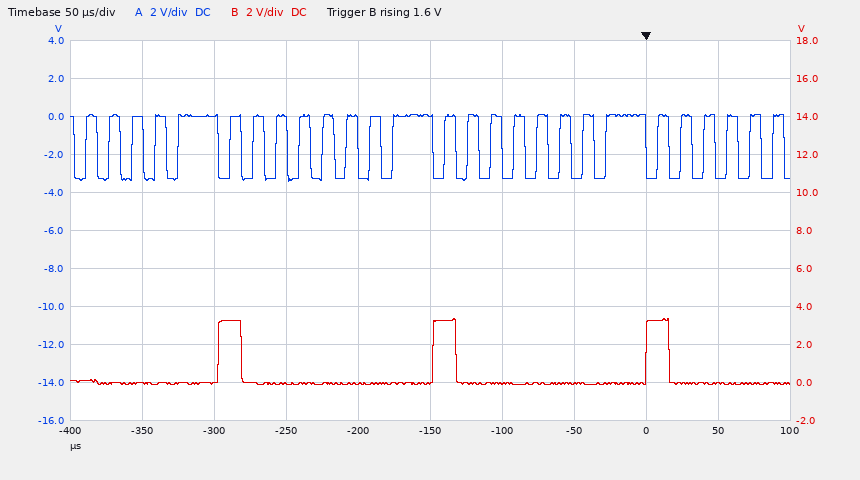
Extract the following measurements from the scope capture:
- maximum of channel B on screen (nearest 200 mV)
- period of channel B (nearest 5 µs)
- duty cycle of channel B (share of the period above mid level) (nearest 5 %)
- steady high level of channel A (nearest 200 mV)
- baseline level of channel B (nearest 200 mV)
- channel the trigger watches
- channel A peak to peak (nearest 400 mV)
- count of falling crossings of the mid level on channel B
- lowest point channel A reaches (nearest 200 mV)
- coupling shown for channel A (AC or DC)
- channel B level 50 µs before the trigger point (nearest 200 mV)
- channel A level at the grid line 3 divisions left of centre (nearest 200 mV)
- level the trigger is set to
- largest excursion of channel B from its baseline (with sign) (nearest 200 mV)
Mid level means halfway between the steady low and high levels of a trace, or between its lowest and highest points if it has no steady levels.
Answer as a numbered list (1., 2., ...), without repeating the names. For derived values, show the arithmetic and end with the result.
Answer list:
1. 3.4 V
2. 150 µs
3. 10 %
4. 0.0 V
5. 0.0 V
6. channel B
7. 3.6 V
8. 3
9. -3.4 V
10. DC
11. 0.0 V
12. 0.0 V
13. 1.6 V
14. 3.4 V − (0.0 V) = +3.4 V
